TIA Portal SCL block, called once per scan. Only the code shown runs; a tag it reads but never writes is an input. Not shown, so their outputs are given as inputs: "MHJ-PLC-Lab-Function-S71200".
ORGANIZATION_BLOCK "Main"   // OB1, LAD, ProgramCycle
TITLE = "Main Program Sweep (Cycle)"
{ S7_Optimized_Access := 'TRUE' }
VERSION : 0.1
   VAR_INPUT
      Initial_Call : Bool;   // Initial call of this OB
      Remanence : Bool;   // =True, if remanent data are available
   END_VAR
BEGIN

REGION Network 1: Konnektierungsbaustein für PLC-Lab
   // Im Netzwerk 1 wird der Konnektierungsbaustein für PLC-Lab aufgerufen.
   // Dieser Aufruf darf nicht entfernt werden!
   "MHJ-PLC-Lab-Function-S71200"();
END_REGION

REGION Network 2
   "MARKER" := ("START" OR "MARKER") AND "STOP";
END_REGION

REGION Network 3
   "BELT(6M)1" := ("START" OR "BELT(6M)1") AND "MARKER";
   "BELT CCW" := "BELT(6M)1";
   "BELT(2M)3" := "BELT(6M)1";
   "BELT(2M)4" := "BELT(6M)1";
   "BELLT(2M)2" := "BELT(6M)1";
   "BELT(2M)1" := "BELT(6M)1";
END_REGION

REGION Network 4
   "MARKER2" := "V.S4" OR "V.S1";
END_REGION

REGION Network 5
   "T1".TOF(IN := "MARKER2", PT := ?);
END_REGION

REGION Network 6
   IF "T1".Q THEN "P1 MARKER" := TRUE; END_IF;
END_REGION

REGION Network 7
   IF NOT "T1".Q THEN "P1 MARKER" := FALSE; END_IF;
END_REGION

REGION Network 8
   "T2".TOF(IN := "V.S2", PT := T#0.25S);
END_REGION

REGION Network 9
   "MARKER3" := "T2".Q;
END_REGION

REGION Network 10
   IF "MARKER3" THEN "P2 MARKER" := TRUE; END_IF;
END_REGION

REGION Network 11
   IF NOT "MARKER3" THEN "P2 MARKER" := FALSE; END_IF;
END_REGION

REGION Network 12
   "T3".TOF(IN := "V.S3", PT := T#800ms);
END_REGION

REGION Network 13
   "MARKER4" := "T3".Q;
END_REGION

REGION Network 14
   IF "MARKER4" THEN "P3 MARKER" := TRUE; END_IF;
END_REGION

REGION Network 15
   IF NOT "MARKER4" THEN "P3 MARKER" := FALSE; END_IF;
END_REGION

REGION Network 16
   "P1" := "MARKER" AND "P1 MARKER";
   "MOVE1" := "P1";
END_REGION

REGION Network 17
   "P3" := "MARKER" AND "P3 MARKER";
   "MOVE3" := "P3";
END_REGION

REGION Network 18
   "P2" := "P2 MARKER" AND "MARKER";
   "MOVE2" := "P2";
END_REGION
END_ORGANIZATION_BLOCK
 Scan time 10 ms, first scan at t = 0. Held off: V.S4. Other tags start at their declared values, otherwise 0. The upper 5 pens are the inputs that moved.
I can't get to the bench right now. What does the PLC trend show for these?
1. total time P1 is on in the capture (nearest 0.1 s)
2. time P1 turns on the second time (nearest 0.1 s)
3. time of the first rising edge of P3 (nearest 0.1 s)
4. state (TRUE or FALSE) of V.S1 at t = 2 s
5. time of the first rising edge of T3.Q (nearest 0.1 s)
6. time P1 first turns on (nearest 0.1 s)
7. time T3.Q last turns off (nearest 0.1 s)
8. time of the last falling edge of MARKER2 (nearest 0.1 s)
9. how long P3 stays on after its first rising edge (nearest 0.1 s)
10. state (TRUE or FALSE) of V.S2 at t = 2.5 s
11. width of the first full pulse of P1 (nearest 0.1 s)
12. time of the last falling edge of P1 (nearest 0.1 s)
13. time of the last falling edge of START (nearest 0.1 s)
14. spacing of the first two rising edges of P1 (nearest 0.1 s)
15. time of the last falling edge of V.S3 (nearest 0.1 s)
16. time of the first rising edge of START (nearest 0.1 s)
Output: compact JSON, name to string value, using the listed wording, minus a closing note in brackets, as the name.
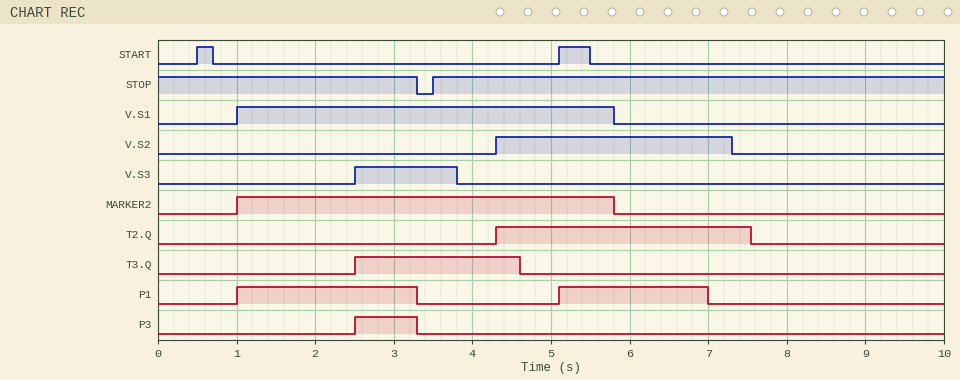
{"total time P1 is on in the capture": "4.2 s", "time P1 turns on the second time": "5.1 s", "time of the first rising edge of P3": "2.5 s", "state (TRUE or FALSE) of V.S1 at t = 2 s": "TRUE", "time of the first rising edge of T3.Q": "2.5 s", "time P1 first turns on": "1.0 s", "time T3.Q last turns off": "4.6 s", "time of the last falling edge of MARKER2": "5.8 s", "how long P3 stays on after its first rising edge": "0.8 s", "state (TRUE or FALSE) of V.S2 at t = 2.5 s": "FALSE", "width of the first full pulse of P1": "2.3 s", "time of the last falling edge of P1": "7.0 s", "time of the last falling edge of START": "5.5 s", "spacing of the first two rising edges of P1": "4.1 s", "time of the last falling edge of V.S3": "3.8 s", "time of the first rising edge of START": "0.5 s"}
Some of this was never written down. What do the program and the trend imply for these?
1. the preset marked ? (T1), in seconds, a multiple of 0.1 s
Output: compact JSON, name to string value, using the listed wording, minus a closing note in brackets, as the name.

{"the preset marked ? (T1), in seconds, a multiple of 0.1 s": "1.2 s"}
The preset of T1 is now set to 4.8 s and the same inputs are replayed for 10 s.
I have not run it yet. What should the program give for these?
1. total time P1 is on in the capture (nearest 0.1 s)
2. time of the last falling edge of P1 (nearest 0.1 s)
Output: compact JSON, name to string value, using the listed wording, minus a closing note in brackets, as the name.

{"total time P1 is on in the capture": "7.2 s", "time of the last falling edge of P1": "3.3 s"}
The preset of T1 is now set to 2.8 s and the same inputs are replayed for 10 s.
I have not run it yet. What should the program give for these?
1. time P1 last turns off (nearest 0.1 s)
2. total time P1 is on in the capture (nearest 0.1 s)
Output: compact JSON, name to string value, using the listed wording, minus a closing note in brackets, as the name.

{"time P1 last turns off": "8.6 s", "total time P1 is on in the capture": "5.8 s"}
